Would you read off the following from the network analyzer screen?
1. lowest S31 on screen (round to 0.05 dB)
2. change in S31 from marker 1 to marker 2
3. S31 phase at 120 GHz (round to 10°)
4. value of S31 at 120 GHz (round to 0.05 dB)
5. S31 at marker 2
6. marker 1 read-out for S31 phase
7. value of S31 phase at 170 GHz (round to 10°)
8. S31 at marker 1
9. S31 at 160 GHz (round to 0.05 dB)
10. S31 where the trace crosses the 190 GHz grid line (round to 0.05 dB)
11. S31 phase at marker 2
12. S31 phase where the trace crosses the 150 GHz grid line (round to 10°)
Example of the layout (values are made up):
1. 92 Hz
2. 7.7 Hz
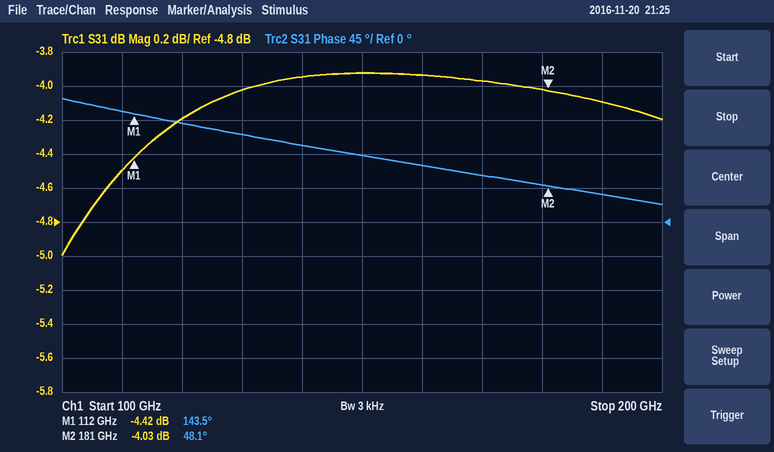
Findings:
1. -5.00 dB
2. 0.39 dB
3. 130°
4. -4.20 dB
5. -4.03 dB
6. 143.5°
7. 60°
8. -4.42 dB
9. -3.95 dB
10. -4.10 dB
11. 48.1°
12. 90°
